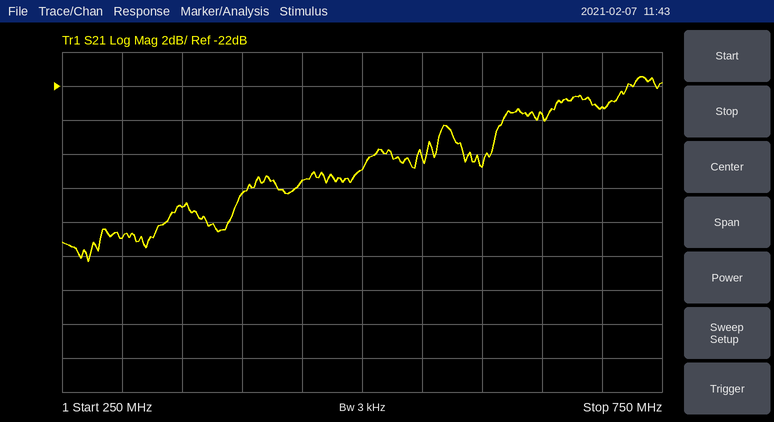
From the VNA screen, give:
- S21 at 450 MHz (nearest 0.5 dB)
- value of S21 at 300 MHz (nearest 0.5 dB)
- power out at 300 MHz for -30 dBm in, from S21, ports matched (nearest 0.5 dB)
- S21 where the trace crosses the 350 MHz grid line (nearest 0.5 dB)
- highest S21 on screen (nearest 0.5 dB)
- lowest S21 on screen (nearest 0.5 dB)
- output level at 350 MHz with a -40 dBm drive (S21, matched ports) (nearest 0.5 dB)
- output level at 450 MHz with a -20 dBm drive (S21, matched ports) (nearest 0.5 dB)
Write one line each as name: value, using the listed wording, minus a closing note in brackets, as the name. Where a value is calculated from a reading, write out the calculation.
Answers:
S21 at 450 MHz: -27.5 dB
value of S21 at 300 MHz: -31.0 dB
power out at 300 MHz for -30 dBm in, from S21, ports matched: -30 dBm + (-31.0 dB) = -61.0 dBm
S21 where the trace crosses the 350 MHz grid line: -29.0 dB
highest S21 on screen: -21.5 dB
lowest S21 on screen: -32.5 dB
output level at 350 MHz with a -40 dBm drive (S21, matched ports): -40 dBm + (-29.0 dB) = -69.0 dBm
output level at 450 MHz with a -20 dBm drive (S21, matched ports): -20 dBm + (-27.5 dB) = -47.5 dBm
